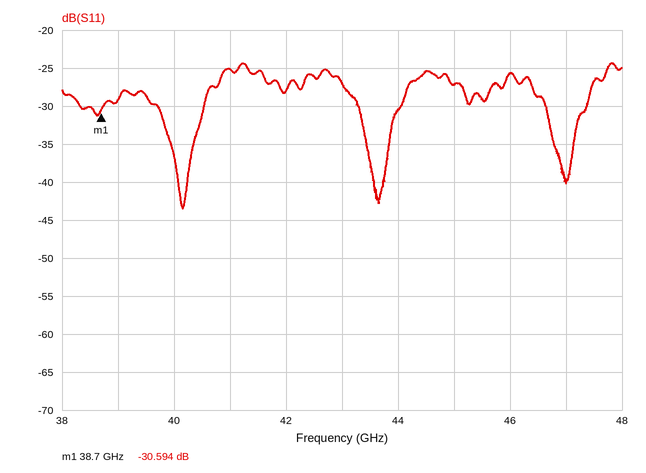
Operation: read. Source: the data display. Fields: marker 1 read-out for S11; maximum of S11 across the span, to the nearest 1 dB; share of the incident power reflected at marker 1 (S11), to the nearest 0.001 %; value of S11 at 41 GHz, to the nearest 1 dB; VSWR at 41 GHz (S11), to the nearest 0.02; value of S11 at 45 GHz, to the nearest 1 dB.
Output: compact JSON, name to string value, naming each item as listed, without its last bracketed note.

{"marker 1 read-out for S11": "-30.594 dB", "maximum of S11 across the span, to the nearest 1 dB": "-24 dB", "share of the incident power reflected at marker 1 (S11), to the nearest 0.001 %": "0.087 %", "value of S11 at 41 GHz, to the nearest 1 dB": "-25 dB", "VSWR at 41 GHz (S11), to the nearest 0.02": "1.12", "value of S11 at 45 GHz, to the nearest 1 dB": "-27 dB"}
